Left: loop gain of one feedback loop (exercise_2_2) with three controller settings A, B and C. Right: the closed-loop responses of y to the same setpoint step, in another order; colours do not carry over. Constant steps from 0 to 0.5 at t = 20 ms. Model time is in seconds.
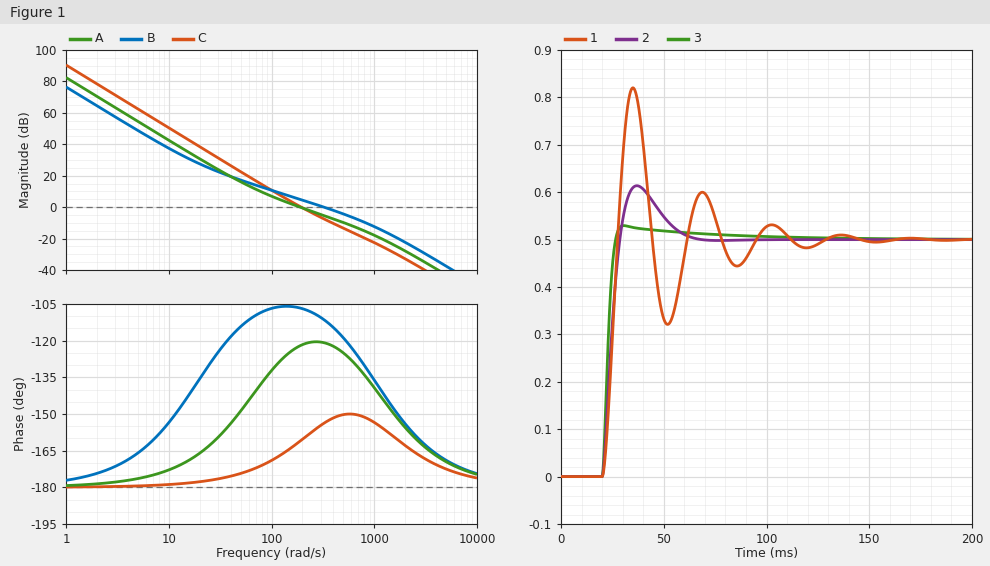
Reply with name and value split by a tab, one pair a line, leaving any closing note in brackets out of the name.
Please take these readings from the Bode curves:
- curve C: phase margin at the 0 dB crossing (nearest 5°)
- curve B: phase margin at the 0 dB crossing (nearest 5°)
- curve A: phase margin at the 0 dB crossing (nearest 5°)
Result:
curve C: phase margin at the 0 dB crossing	20°
curve B: phase margin at the 0 dB crossing	70°
curve A: phase margin at the 0 dB crossing	60°
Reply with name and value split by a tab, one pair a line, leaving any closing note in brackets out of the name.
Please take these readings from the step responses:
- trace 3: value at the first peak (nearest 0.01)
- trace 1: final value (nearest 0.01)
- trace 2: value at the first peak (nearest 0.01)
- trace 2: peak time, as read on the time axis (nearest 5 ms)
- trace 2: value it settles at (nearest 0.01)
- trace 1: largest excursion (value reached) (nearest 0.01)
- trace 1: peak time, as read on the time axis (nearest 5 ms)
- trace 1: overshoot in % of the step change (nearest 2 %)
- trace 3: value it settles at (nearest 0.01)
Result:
trace 3: value at the first peak	0.53
trace 1: final value	0.50
trace 2: value at the first peak	0.61
trace 2: peak time, as read on the time axis	35 ms
trace 2: value it settles at	0.50
trace 1: largest excursion (value reached)	0.82
trace 1: peak time, as read on the time axis	35 ms
trace 1: overshoot in % of the step change	64 %
trace 3: value it settles at	0.50
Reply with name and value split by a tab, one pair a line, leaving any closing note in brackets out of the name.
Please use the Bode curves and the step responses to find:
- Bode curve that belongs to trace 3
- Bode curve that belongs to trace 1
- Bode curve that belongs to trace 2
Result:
Bode curve that belongs to trace 3	B
Bode curve that belongs to trace 1	C
Bode curve that belongs to trace 2	A
